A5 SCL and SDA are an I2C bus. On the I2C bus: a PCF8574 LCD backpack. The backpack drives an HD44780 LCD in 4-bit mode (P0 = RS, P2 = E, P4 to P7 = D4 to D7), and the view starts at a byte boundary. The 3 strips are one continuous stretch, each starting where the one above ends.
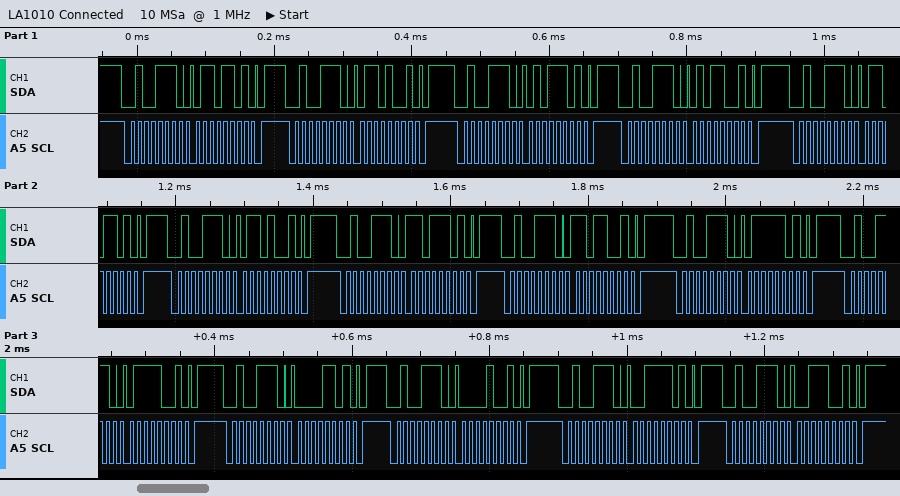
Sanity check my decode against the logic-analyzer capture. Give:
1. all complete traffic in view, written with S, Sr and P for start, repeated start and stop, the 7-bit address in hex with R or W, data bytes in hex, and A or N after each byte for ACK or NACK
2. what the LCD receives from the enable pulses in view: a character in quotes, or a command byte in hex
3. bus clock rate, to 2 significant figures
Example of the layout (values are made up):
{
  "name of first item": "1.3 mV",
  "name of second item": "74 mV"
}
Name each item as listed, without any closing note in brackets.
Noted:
{
  "all complete traffic in view, written with S, Sr and P for start, repeated start and stop, the 7-bit address in hex with R or W, data bytes in hex, and A or N after each byte for ACK or NACK": "S 27W A 6D A P S 27W A 69 A P S 27W A 5D A P S 27W A 59 A P S 27W A 6D A P S 27W A 69 A P S 27W A DD A P S 27W A D9 A P S 27W A 7D A P S 27W A 79 A P S 27W A 0D A P S 27W A 09 A P S 27W A 3D A P S 27W A 39 A P",
  "what the LCD receives from the enable pulses in view: a character in quotes, or a command byte in hex": "'e' 'm' 'p'",
  "bus clock rate, to 2 significant figures": "100 kHz"
}
